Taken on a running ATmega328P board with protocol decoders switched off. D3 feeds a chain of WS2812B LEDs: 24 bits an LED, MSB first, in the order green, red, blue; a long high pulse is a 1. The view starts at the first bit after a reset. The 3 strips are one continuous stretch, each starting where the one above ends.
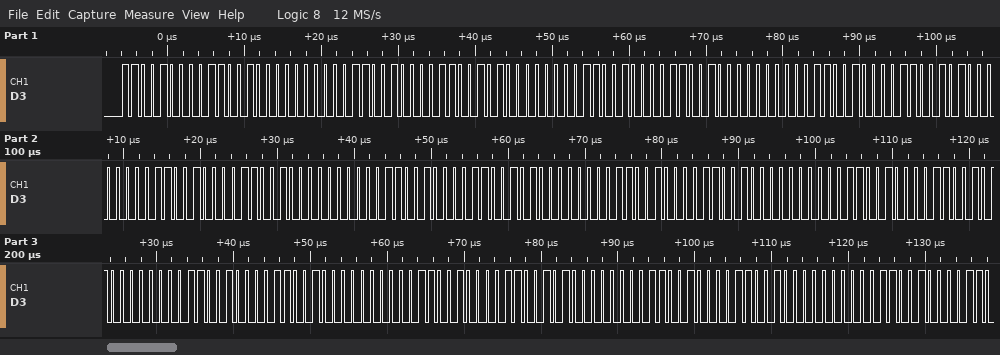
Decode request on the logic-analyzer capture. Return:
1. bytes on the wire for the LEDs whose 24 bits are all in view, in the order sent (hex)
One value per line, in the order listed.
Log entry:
C8 64 00 C8 65 00 C8 64 00 C8 65 00 C8 64 00 C8 65 00 C8 64 00 C8 65 00 C8 64 00 C8 65 00 C8 64 00
